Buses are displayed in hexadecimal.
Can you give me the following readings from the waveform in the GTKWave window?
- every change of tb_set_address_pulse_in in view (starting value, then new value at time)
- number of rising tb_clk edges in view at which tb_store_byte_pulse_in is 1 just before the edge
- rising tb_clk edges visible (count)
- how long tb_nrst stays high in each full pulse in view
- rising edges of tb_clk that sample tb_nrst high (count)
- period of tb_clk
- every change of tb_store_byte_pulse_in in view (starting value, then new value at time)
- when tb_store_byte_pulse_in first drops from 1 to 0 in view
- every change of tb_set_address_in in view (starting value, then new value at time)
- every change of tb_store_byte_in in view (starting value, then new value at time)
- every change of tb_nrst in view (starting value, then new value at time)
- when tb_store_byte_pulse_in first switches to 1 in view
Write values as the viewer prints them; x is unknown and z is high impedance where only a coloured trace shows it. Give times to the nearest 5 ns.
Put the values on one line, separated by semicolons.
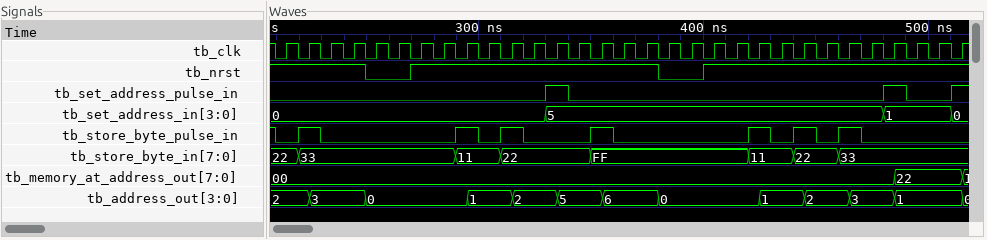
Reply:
0, 1 at 330 ns, 0 at 340 ns, 1 at 480 ns, 0 at 490 ns, 1 at 510 ns; 7; 31; 110 ns; 27; 10 ns; 1, 0 at 210 ns, 1 at 220 ns, 0 at 230 ns, 1 at 290 ns, 0 at 300 ns, 1 at 310 ns, 0 at 320 ns, 1 at 350 ns, 0 at 360 ns, 1 at 420 ns, 0 at 430 ns, 1 at 440 ns, 0 at 450 ns, 1 at 460 ns, 0 at 470 ns; 210 ns; 0, 5 at 330 ns, 1 at 480 ns, 0 at 510 ns; 22, 33 at 220 ns, 11 at 290 ns, 22 at 310 ns, FF at 350 ns, 11 at 420 ns, 22 at 440 ns, 33 at 460 ns; 1, 0 at 250 ns, 1 at 270 ns, 0 at 380 ns, 1 at 400 ns; 220 ns
